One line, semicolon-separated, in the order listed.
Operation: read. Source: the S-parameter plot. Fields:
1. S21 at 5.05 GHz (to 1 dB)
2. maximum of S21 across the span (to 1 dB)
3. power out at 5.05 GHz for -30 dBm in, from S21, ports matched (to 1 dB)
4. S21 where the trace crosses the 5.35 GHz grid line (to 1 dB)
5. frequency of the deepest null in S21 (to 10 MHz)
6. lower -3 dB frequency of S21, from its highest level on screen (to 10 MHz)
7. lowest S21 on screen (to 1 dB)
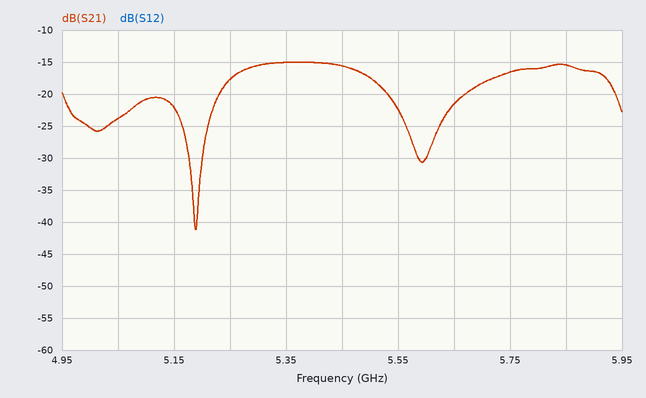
-24 dB; -15 dB; -54 dBm; -15 dB; 5.19 GHz; 5.25 GHz; -41 dB
